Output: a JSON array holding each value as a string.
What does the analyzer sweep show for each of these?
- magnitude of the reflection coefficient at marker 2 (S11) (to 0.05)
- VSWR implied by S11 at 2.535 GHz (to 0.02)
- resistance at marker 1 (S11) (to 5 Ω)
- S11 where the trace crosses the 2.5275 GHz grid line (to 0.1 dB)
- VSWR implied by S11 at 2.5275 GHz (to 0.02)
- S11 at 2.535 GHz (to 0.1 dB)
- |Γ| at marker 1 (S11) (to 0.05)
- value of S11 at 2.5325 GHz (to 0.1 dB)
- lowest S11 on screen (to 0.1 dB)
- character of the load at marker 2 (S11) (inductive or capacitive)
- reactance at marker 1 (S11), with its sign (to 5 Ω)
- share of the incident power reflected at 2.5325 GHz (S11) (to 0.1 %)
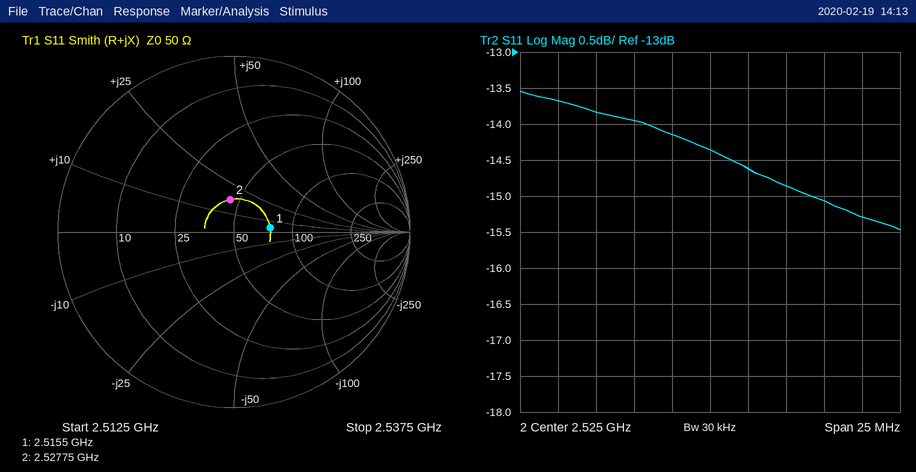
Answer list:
["0.20", "1.42", "75 Ω", "-14.6 dB", "1.46", "-15.3 dB", "0.20", "-15.1 dB", "-15.5 dB", "inductive", "+5 Ω", "3.1 %"]
